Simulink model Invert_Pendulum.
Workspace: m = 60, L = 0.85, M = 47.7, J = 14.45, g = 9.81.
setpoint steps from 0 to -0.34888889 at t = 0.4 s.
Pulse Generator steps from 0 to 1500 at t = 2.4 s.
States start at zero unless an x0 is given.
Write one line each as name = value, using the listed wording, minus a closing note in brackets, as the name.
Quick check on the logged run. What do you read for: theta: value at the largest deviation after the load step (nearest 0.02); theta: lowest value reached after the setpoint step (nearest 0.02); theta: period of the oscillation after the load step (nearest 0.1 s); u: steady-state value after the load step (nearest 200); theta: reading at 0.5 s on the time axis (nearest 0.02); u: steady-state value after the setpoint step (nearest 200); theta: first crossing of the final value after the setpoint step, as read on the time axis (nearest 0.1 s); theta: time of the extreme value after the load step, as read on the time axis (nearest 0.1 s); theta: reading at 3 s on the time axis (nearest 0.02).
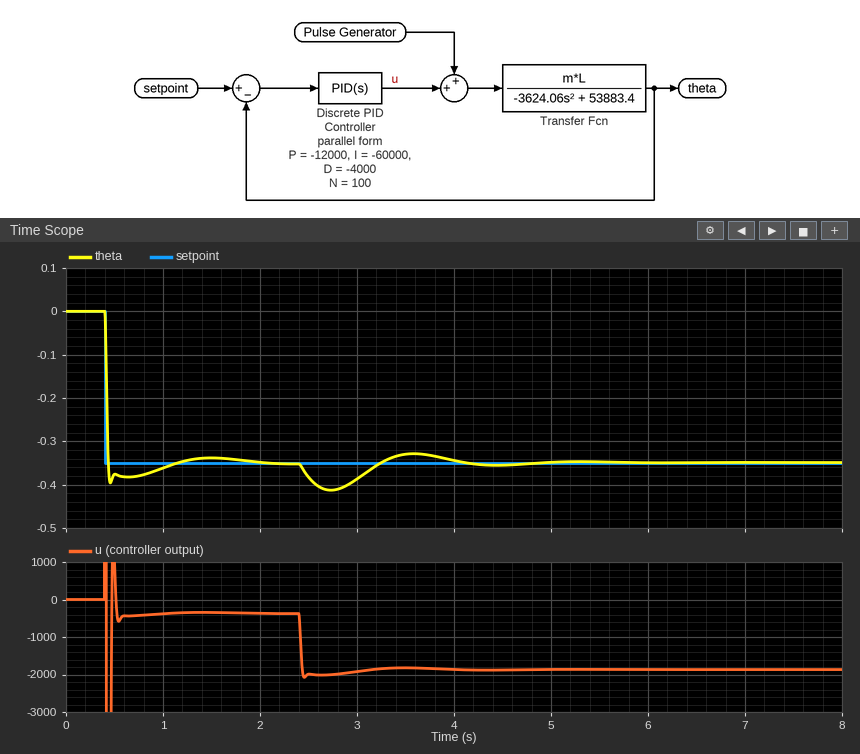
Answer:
theta: value at the largest deviation after the load step = -0.42
theta: lowest value reached after the setpoint step = -0.40
theta: period of the oscillation after the load step = 1.7 s
u: steady-state value after the load step = -1800
theta: reading at 0.5 s on the time axis = -0.38
u: steady-state value after the setpoint step = -400
theta: first crossing of the final value after the setpoint step, as read on the time axis = 0.4 s
theta: time of the extreme value after the load step, as read on the time axis = 2.7 s
theta: reading at 3 s on the time axis = -0.38
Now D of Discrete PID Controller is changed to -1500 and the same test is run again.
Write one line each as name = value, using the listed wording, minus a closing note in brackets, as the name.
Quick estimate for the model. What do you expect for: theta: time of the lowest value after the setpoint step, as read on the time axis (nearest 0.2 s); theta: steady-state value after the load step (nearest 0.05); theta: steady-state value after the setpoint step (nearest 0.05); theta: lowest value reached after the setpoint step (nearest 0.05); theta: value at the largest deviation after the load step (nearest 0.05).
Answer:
theta: time of the lowest value after the setpoint step, as read on the time axis = 0.6 s
theta: steady-state value after the load step = -0.35
theta: steady-state value after the setpoint step = -0.35
theta: lowest value reached after the setpoint step = -0.45
theta: value at the largest deviation after the load step = -0.45
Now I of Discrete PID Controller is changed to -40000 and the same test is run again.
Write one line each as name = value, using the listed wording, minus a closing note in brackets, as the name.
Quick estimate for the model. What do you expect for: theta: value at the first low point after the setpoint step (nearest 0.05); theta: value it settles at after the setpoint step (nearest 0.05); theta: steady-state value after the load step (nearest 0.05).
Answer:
theta: value at the first low point after the setpoint step = -0.40
theta: value it settles at after the setpoint step = -0.35
theta: steady-state value after the load step = -0.35
